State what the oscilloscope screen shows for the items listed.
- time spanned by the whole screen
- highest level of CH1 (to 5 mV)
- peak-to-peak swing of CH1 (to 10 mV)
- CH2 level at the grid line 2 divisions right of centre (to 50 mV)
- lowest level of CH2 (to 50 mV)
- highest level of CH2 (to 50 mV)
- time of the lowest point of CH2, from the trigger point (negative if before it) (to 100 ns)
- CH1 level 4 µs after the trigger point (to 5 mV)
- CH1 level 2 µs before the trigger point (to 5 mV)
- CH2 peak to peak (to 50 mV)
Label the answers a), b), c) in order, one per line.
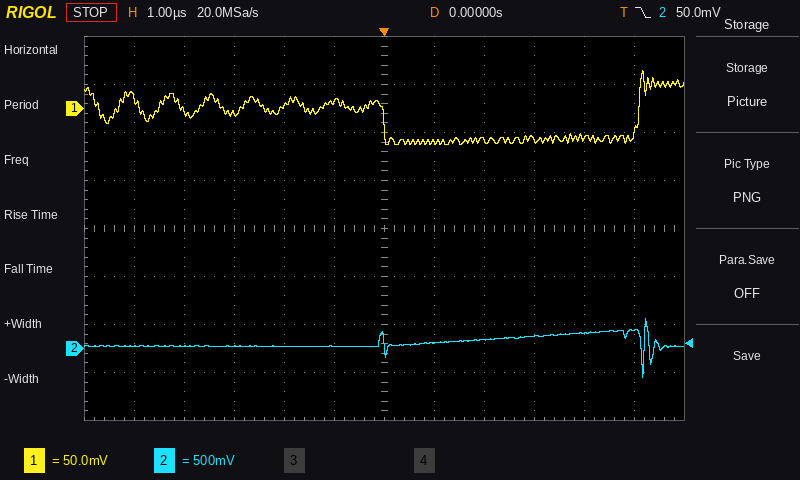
a) 12 µs
b) 40 mV
c) 80 mV
d) 100 mV
e) -300 mV
f) 300 mV
g) +5.2 µs
h) -30 mV
i) 5 mV
j) 600 mV
